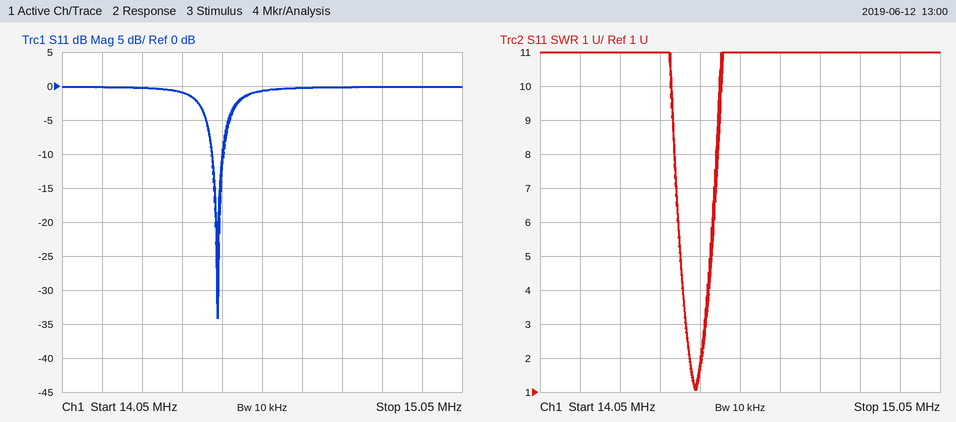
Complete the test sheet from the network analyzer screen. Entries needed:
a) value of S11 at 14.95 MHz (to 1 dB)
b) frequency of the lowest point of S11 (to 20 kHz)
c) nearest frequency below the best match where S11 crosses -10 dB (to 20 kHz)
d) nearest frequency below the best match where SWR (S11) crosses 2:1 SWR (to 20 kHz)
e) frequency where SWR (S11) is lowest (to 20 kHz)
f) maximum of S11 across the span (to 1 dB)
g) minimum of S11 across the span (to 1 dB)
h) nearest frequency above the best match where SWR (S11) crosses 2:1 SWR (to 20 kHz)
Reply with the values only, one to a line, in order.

0 dB
14.44 MHz
14.42 MHz
14.42 MHz
14.44 MHz
0 dB
-34 dB
14.46 MHz
